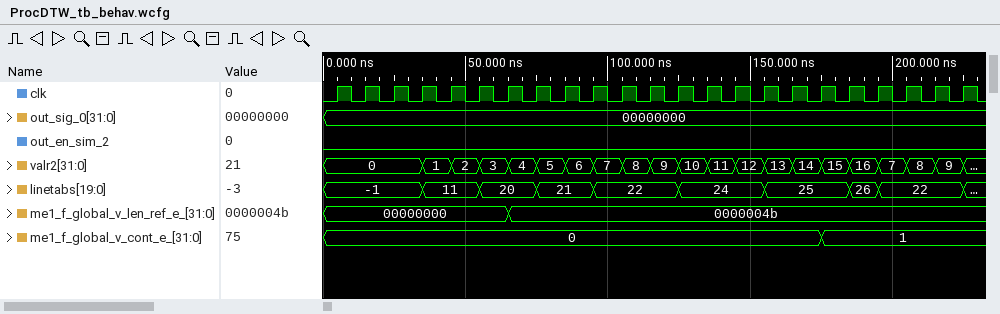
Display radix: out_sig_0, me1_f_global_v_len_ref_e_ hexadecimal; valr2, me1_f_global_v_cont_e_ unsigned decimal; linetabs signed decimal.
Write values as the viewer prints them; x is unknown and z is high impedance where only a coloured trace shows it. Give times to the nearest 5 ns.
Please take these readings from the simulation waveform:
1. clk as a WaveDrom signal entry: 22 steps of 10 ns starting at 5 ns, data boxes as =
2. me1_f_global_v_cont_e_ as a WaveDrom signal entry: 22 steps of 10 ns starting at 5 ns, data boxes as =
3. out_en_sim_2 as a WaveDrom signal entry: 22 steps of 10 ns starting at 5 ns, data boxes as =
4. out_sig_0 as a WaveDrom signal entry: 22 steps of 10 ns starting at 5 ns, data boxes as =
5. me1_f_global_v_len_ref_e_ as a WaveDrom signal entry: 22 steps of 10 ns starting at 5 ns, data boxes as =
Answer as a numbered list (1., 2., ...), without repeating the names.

1. {name: 'clk', wave: 'p.....................'}
2. {name: 'me1_f_global_v_cont_e_', wave: '=................=....', data: '0 1'}
3. {name: 'out_en_sim_2', wave: '0.....................'}
4. {name: 'out_sig_0', wave: '=.....................', data: '00000000'}
5. {name: 'me1_f_global_v_len_ref_e_', wave: '=.....=...............', data: '00000000 0000004b'}
